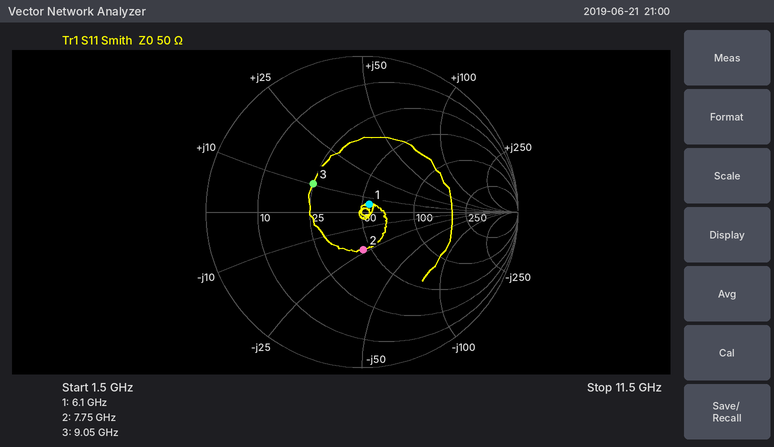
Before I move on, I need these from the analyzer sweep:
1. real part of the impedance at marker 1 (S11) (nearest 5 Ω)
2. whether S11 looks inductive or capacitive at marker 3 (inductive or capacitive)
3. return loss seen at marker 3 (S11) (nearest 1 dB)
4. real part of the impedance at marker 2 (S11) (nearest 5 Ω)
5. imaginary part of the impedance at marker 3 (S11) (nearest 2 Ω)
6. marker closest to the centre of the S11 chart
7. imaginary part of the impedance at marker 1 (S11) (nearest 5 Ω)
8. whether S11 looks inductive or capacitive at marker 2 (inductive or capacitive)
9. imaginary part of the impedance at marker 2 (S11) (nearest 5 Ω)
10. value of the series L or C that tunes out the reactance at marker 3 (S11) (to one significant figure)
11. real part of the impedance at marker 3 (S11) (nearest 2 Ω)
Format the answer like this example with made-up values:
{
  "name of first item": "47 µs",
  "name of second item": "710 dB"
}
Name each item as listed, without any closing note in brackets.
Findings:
{
  "real part of the impedance at marker 1 (S11)": "55 Ω",
  "whether S11 looks inductive or capacitive at marker 3": "inductive",
  "return loss seen at marker 3 (S11)": "9 dB",
  "real part of the impedance at marker 2 (S11)": "45 Ω",
  "imaginary part of the impedance at marker 3 (S11)": "+10 Ω",
  "marker closest to the centre of the S11 chart": "marker 1",
  "imaginary part of the impedance at marker 1 (S11)": "+5 Ω",
  "whether S11 looks inductive or capacitive at marker 2": "capacitive",
  "imaginary part of the impedance at marker 2 (S11)": "-25 Ω",
  "value of the series L or C that tunes out the reactance at marker 3 (S11)": "2 pF",
  "real part of the impedance at marker 3 (S11)": "24 Ω"
}
